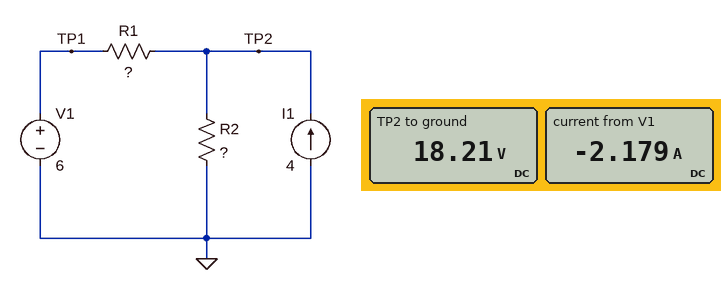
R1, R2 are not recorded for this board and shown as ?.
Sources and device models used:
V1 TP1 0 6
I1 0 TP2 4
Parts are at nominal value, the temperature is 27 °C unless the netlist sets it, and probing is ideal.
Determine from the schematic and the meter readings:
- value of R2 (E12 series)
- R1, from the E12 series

10 Ω
5.6 Ω
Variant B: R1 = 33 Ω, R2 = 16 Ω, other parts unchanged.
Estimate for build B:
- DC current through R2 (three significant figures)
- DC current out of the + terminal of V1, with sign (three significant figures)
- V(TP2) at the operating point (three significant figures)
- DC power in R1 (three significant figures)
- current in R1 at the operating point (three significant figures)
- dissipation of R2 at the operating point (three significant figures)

2.82 A
-1.18 A
45.1 V
46.2 W
1.18 A
127 W
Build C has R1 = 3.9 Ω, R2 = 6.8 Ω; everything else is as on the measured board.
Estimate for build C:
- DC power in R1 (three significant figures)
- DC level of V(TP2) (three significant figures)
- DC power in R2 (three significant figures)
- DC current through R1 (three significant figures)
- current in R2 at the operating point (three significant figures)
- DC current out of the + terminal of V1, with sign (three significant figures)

15.3 W
13.7 V
27.7 W
1.98 A
2.02 A
-1.98 A
